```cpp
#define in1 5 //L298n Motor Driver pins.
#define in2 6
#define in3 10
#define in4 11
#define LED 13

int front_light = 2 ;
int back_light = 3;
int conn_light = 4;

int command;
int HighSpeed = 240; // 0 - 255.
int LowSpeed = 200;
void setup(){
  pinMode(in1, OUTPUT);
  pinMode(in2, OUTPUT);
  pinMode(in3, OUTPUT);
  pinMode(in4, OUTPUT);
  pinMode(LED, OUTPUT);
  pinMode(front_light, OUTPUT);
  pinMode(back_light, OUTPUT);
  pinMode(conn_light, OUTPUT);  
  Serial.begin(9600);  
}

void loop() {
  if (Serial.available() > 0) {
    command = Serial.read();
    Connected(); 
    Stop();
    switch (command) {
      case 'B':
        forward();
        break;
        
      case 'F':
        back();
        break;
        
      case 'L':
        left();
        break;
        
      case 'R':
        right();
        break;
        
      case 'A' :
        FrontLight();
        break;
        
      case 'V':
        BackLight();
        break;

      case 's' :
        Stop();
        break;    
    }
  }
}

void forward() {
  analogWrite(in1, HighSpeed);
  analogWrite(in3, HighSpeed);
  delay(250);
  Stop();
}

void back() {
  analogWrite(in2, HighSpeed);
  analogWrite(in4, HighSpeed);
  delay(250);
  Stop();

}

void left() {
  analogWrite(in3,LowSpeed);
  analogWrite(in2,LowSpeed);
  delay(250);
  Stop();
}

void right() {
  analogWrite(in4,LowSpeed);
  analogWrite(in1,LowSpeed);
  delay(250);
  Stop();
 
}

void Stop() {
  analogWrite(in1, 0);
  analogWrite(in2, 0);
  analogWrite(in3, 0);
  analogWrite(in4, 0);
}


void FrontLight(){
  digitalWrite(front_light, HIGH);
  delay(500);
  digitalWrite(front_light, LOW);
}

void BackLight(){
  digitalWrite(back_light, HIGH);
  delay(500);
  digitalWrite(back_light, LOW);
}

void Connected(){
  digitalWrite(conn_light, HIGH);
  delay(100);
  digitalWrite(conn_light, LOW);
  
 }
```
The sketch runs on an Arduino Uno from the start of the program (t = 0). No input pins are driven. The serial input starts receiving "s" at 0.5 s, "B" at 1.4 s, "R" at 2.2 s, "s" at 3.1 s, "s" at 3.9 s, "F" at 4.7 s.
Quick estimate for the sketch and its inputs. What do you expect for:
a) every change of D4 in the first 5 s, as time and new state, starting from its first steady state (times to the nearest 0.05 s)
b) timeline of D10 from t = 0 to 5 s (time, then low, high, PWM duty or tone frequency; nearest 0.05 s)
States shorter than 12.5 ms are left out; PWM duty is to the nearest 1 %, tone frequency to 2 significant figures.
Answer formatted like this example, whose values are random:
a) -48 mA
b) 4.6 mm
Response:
a) 0 s low; 0.5 s high; 0.6 s low; 1.4 s high; 1.5 s low; 2.2 s high; 2.3 s low; 3.1 s high; 3.2 s low; 3.9 s high; 4 s low; 4.7 s high; 4.8 s low
b) 0 s low; 1.5 s PWM 94 %; 1.75 s low
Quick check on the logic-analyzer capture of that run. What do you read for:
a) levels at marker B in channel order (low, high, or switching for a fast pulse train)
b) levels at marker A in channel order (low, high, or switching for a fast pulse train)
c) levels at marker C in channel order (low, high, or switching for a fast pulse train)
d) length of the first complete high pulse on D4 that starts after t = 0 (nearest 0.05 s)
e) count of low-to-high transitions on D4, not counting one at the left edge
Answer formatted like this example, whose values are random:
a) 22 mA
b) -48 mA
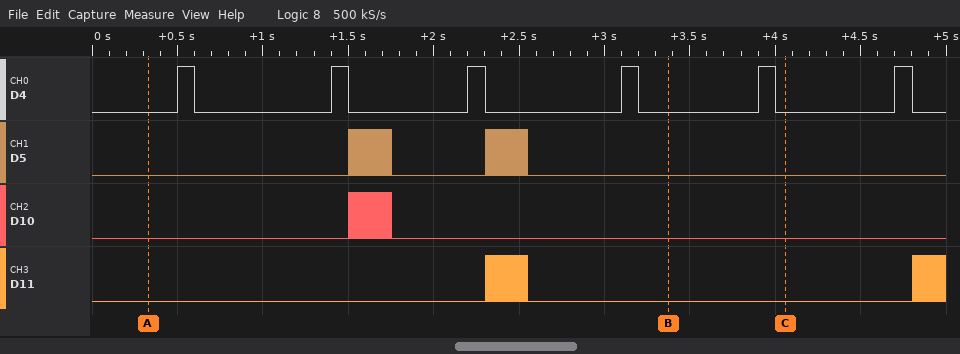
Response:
a) D4 low, D5 low, D10 low, D11 low
b) D4 low, D5 low, D10 low, D11 low
c) D4 low, D5 low, D10 low, D11 low
d) 0.10 s
e) 6
